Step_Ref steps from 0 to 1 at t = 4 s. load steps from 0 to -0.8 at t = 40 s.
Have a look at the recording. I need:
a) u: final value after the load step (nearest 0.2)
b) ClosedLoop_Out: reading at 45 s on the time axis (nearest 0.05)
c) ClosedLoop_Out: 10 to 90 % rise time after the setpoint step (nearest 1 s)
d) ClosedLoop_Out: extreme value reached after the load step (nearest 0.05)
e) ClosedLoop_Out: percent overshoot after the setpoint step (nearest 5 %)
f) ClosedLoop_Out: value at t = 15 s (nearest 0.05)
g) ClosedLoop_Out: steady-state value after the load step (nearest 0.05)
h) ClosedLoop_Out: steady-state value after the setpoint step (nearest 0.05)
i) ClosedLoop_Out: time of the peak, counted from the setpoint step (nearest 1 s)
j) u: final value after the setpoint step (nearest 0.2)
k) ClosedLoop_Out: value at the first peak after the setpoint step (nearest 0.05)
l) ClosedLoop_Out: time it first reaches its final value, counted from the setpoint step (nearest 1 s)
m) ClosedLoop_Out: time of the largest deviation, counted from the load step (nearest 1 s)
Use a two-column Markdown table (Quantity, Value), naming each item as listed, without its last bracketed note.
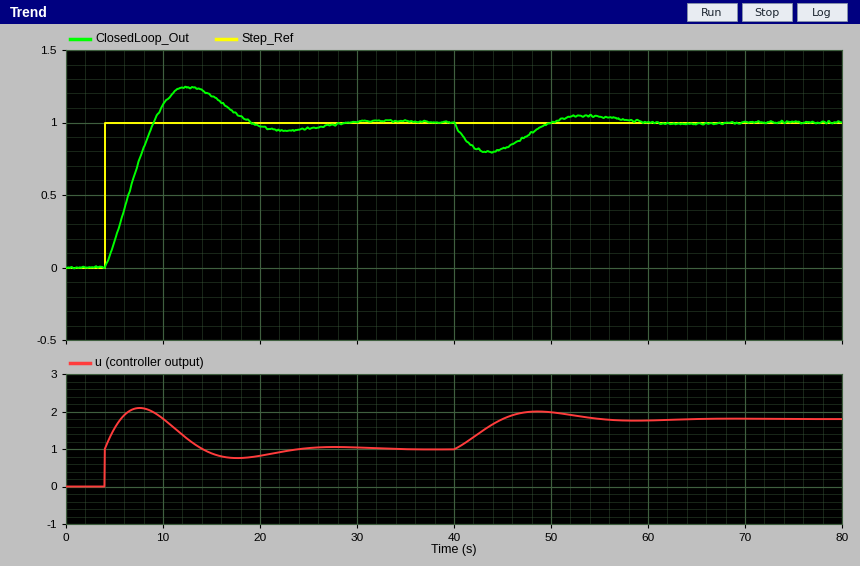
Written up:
| Quantity | Value |
|---|---|
| u: final value after the load step | 1.8 |
| ClosedLoop_Out: reading at 45 s on the time axis | 0.80 |
| ClosedLoop_Out: 10 to 90 % rise time after the setpoint step | 4 s |
| ClosedLoop_Out: extreme value reached after the load step | 0.80 |
| ClosedLoop_Out: percent overshoot after the setpoint step | 25 % |
| ClosedLoop_Out: value at t = 15 s | 1.20 |
| ClosedLoop_Out: steady-state value after the load step | 1.00 |
| ClosedLoop_Out: steady-state value after the setpoint step | 1.00 |
| ClosedLoop_Out: time of the peak, counted from the setpoint step | 9 s |
| u: final value after the setpoint step | 1.0 |
| ClosedLoop_Out: value at the first peak after the setpoint step | 1.25 |
| ClosedLoop_Out: time it first reaches its final value, counted from the setpoint step | 5 s |
| ClosedLoop_Out: time of the largest deviation, counted from the load step | 4 s |
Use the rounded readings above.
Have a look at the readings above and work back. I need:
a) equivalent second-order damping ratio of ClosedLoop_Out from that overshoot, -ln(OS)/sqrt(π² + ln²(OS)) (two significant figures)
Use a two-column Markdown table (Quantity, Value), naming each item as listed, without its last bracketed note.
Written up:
| Quantity | Value |
|---|---|
| equivalent second-order damping ratio of ClosedLoop_Out from that overshoot, -ln(OS)/sqrt(π² + ln²(OS)) | 0.40 |
